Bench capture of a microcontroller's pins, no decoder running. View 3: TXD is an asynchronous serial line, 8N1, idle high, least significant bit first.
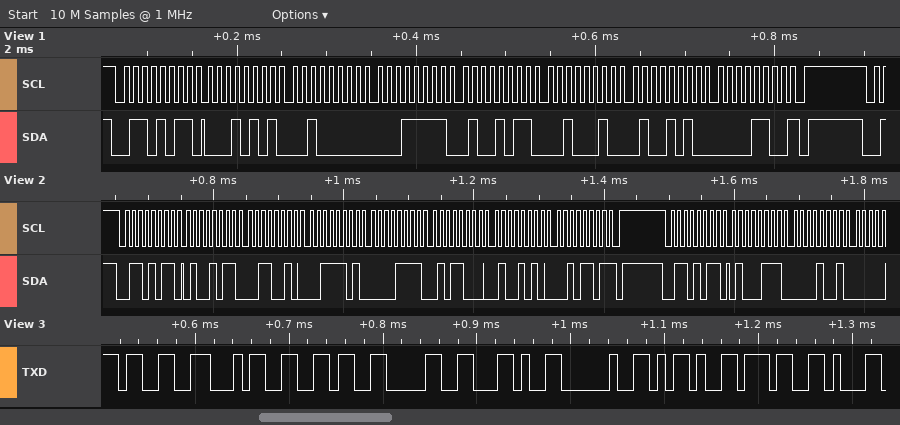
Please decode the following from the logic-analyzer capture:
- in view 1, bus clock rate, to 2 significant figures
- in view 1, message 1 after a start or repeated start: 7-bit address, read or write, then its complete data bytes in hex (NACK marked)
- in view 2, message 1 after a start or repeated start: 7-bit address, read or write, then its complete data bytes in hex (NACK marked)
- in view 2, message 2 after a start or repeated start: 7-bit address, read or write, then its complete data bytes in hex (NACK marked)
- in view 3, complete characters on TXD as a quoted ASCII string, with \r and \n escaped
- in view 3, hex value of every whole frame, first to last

100 kHz
0x35 read: 15 20 1F 4B 22 4A 0C NACK
0x35 read: 4B 32 3D 0F 58 4A 2D NACK
0x35 read: 47 09
"3460, -7"
0x33 0x34 0x36 0x30 0x2C 0x20 0x2D 0x37
